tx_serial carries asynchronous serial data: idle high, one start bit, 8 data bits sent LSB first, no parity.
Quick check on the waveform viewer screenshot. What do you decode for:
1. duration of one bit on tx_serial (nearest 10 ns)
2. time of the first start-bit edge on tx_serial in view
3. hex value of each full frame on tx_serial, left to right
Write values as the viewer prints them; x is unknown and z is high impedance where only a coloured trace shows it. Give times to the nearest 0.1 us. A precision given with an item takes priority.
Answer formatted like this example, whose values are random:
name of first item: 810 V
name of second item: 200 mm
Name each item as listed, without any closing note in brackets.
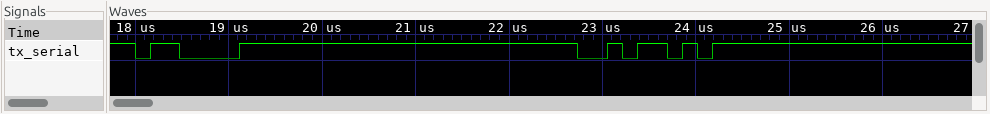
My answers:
duration of one bit on tx_serial: 160 ns
time of the first start-bit edge on tx_serial in view: 18 us
hex value of each full frame on tx_serial, left to right: C3, 5A
